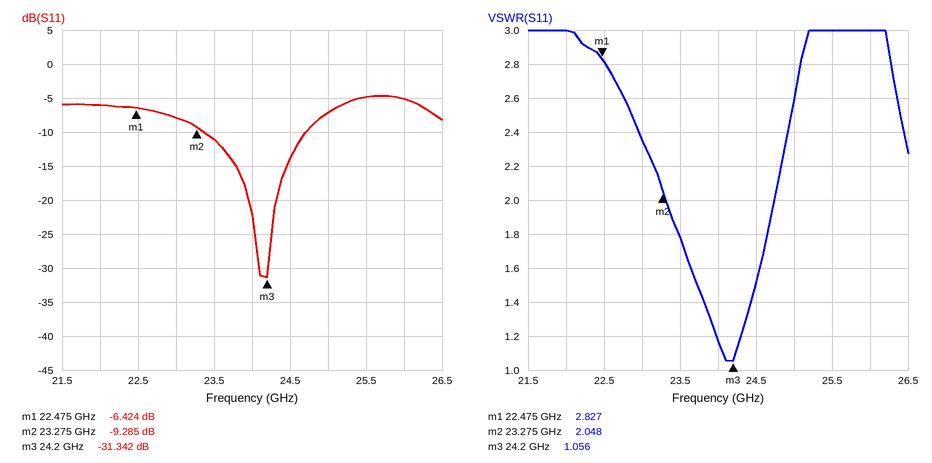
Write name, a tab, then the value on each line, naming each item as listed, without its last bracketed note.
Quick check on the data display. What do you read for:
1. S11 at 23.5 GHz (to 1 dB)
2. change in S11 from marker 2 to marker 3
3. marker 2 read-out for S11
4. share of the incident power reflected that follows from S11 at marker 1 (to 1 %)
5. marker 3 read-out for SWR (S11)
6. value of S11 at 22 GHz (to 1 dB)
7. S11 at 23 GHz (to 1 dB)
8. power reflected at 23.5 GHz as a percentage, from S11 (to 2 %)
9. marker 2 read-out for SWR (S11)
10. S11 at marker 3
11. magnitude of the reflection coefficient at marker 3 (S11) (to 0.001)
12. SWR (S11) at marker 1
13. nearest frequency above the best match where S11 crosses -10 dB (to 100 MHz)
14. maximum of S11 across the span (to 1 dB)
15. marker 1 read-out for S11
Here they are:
S11 at 23.5 GHz	-11 dB
change in S11 from marker 2 to marker 3	-22.057 dB
marker 2 read-out for S11	-9.285 dB
share of the incident power reflected that follows from S11 at marker 1	23 %
marker 3 read-out for SWR	1.056
value of S11 at 22 GHz	-6 dB
S11 at 23 GHz	-8 dB
power reflected at 23.5 GHz as a percentage, from S11	8 %
marker 2 read-out for SWR	2.048
S11 at marker 3	-31.342 dB
magnitude of the reflection coefficient at marker 3 (S11)	0.027
SWR (S11) at marker 1	2.827
nearest frequency above the best match where S11 crosses -10 dB	24.7 GHz
maximum of S11 across the span	-5 dB
marker 1 read-out for S11	-6.424 dB
